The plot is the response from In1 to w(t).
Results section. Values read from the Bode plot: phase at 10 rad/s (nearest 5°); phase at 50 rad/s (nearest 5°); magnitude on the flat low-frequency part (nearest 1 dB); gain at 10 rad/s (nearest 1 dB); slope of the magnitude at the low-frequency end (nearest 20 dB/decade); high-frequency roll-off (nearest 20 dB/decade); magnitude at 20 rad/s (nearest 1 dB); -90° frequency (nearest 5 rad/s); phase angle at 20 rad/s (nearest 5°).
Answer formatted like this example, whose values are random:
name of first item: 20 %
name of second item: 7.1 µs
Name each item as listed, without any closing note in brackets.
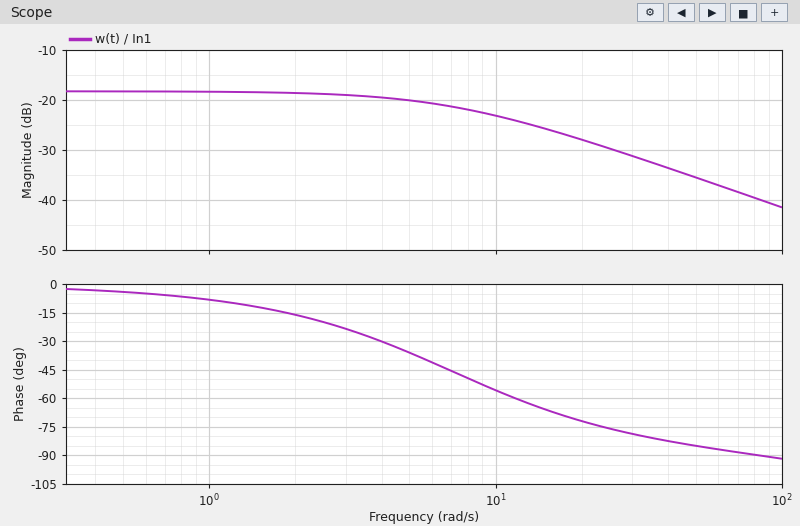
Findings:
phase at 10 rad/s: -55°
phase at 50 rad/s: -85°
magnitude on the flat low-frequency part: -18 dB
gain at 10 rad/s: -23 dB
slope of the magnitude at the low-frequency end: 0 dB/decade
high-frequency roll-off: -20 dB/decade
magnitude at 20 rad/s: -28 dB
-90° frequency: 85 rad/s
phase angle at 20 rad/s: -70°
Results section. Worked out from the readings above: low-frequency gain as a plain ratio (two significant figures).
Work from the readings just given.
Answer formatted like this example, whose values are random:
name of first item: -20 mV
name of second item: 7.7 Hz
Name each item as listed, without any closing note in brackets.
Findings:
low-frequency gain as a plain ratio: 0.13
